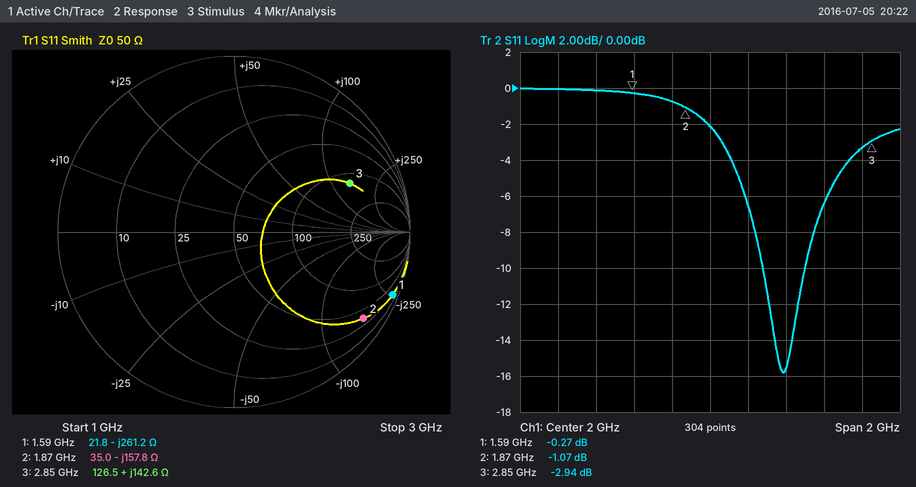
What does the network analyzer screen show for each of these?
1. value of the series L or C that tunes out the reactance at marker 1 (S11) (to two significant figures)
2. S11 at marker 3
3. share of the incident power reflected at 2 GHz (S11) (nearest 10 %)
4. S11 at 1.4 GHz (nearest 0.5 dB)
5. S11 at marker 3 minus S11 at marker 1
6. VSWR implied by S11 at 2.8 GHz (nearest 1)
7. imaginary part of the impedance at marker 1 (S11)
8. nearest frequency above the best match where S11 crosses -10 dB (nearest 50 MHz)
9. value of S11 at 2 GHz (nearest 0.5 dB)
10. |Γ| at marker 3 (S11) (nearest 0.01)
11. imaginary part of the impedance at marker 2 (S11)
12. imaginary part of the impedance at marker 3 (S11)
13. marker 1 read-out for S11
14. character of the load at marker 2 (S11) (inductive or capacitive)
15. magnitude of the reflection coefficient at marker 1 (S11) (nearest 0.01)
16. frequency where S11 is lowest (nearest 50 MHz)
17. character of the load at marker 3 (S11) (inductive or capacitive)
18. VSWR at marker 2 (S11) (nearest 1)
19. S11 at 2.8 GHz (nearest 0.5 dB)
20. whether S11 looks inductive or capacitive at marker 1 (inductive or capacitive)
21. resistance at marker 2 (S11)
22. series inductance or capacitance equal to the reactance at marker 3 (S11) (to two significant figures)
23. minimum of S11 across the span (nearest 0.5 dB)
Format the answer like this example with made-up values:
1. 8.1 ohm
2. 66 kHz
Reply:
1. 26 nH
2. -2.94 dB
3. 60 %
4. 0.0 dB
5. -2.67 dB
6. 5
7. -261.2 Ω
8. 2.50 GHz
9. -2.0 dB
10. 0.71
11. -157.8 Ω
12. +142.6 Ω
13. -0.27 dB
14. capacitive
15. 0.97
16. 2.40 GHz
17. inductive
18. 16
19. -3.5 dB
20. capacitive
21. 35.0 Ω
22. 8.0 nH
23. -16.0 dB
